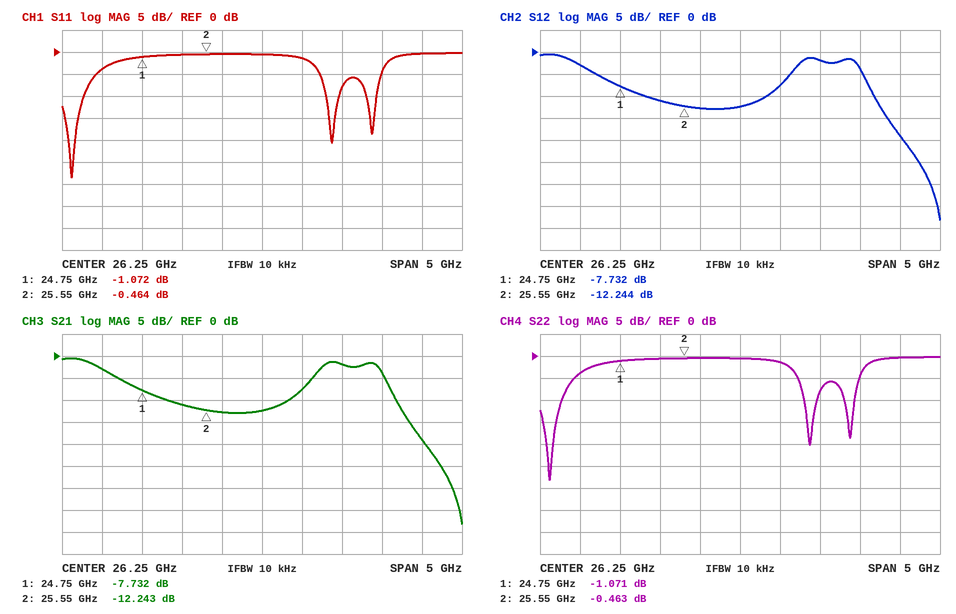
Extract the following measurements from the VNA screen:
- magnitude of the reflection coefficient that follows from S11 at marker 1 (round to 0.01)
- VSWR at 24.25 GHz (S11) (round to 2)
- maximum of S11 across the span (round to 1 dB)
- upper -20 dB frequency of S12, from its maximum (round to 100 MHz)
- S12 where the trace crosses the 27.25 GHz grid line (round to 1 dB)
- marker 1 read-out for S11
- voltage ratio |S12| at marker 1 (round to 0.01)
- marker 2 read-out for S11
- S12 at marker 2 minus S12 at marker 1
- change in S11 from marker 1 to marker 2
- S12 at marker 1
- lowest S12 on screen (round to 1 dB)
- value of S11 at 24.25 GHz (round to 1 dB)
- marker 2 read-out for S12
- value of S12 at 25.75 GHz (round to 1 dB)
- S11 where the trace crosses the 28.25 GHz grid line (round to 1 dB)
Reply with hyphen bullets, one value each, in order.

- 0.88
- 4
- 0 dB
- 28.3 GHz
- -2 dB
- -1.072 dB
- 0.41
- -0.464 dB
- -4.512 dB
- 0.608 dB
- -7.732 dB
- -38 dB
- -4 dB
- -12.244 dB
- -13 dB
- 0 dB
